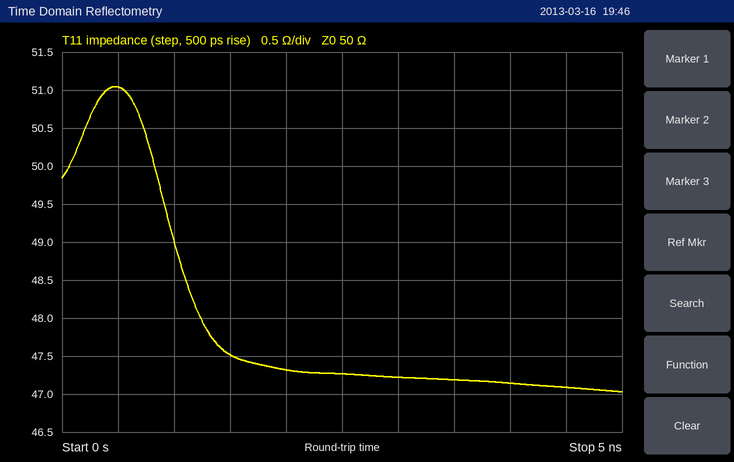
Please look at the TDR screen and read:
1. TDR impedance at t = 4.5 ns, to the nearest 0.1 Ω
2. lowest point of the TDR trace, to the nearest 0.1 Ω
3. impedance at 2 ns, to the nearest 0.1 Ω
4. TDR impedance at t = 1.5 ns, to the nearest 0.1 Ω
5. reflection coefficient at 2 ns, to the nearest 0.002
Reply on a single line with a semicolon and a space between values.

47.1 Ω; 47.0 Ω; 47.3 Ω; 47.5 Ω; -0.028
